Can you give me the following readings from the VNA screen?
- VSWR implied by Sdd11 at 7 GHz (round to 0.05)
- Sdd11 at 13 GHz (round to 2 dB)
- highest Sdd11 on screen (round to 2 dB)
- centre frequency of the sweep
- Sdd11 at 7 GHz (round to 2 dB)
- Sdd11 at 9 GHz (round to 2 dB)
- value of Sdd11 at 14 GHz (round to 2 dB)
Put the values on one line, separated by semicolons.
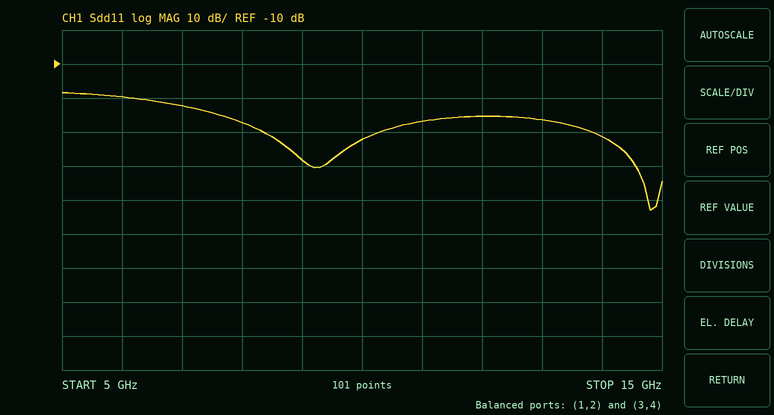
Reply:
1.15; -26 dB; -18 dB; 10 GHz; -22 dB; -38 dB; -32 dB
